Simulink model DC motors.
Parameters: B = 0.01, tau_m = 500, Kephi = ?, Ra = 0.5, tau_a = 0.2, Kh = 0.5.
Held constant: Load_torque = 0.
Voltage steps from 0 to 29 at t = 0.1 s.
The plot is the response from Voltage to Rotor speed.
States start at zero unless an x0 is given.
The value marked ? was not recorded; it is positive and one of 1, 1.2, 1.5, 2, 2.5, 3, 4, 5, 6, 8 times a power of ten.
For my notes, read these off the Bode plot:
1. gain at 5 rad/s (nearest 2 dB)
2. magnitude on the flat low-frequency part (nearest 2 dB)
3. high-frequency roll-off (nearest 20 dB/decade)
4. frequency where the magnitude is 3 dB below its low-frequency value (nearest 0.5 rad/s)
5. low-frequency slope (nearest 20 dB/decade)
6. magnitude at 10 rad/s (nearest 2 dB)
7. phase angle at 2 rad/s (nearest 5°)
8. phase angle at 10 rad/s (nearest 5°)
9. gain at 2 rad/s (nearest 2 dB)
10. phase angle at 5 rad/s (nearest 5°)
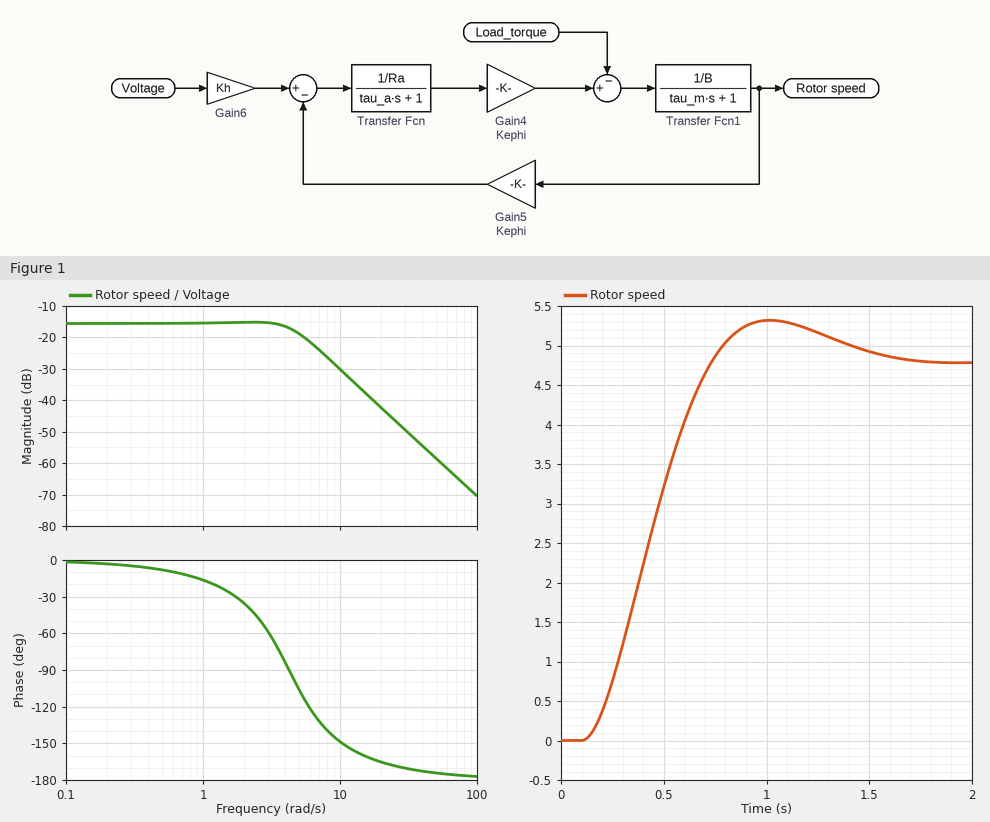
-18 dB
-16 dB
-40 dB/decade
5.0 rad/s
0 dB/decade
-30 dB
-35°
-150°
-16 dB
-105°
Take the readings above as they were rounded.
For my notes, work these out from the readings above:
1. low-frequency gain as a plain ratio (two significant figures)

0.16
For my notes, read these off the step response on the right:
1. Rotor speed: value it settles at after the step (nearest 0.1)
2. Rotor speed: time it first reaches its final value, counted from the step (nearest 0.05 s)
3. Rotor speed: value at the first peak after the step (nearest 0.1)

4.8
0.65 s
5.3
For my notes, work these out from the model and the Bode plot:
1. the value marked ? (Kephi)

3
